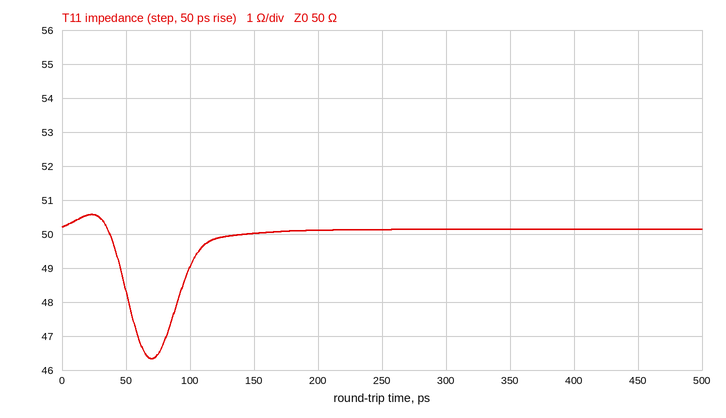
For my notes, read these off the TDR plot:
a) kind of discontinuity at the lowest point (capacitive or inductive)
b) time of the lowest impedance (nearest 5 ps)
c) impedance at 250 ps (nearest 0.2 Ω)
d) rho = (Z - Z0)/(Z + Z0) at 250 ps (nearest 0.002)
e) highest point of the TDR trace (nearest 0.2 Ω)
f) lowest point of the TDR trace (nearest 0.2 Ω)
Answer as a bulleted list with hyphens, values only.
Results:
- capacitive
- 70 ps
- 50.2 Ω
- +0.002
- 50.6 Ω
- 46.4 Ω
